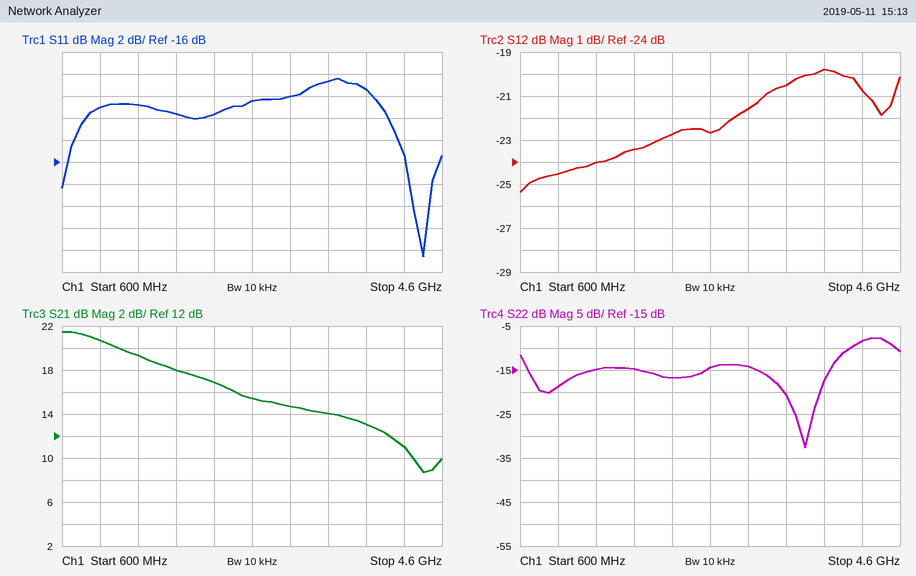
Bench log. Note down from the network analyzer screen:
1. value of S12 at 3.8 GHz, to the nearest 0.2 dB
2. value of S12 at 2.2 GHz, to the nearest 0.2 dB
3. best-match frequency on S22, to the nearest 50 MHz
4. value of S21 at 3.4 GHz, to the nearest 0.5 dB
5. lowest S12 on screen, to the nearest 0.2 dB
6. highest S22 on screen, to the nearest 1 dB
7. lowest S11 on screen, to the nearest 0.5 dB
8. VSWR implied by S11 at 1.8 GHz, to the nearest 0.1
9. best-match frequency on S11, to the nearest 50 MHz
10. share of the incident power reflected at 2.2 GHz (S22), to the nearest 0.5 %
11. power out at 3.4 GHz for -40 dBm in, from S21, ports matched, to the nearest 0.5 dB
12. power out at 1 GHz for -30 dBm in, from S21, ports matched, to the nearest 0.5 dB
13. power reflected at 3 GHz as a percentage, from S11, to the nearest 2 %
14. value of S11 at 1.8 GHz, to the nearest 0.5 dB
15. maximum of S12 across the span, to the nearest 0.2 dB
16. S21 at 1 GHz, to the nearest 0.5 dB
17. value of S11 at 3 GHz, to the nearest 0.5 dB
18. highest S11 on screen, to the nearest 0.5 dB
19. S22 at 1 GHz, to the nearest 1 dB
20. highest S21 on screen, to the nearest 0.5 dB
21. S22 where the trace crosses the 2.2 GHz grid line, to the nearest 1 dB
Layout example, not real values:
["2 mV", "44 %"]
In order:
["-19.8 dB", "-22.8 dB", "3.60 GHz", "14.0 dB", "-25.4 dB", "-8 dB", "-24.5 dB", "1.7", "4.40 GHz", "2.0 %", "-26.0 dBm", "-9.5 dBm", "10 %", "-11.5 dB", "-19.8 dB", "20.5 dB", "-10.0 dB", "-8.5 dB", "-19 dB", "21.5 dB", "-17 dB"]
